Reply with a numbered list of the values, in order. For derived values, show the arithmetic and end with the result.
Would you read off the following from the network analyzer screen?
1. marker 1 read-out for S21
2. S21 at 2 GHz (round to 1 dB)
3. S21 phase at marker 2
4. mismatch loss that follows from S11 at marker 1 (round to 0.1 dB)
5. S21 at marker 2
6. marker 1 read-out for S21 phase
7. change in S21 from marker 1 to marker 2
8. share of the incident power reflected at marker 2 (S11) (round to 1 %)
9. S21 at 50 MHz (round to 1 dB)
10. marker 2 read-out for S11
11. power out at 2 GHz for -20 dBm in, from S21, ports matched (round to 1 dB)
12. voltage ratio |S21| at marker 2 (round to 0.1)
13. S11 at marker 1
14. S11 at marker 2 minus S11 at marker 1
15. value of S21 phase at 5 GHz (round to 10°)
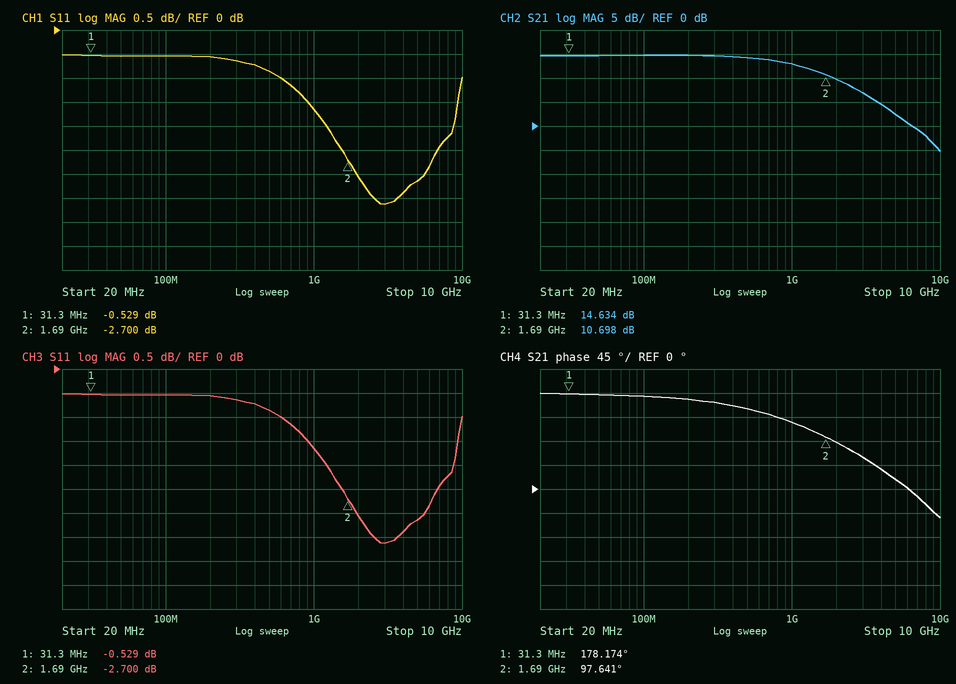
1. 14.634 dB
2. 10 dB
3. 97.641°
4. −10 log10(1 − 10^(-0.529/10)) ≈ 9.4 dB
5. 10.698 dB
6. 178.174°
7. 10.698 − (14.634) = -3.936 dB
8. 10^(-2.7/10) ≈ 54 %
9. 15 dB
10. -2.700 dB
11. -20 dBm + (10 dB) = -10 dBm
12. 10^(10.698/20) ≈ 3.4
13. -0.529 dB
14. -2.7 − (-0.529) = -2.171 dB
15. 20°
